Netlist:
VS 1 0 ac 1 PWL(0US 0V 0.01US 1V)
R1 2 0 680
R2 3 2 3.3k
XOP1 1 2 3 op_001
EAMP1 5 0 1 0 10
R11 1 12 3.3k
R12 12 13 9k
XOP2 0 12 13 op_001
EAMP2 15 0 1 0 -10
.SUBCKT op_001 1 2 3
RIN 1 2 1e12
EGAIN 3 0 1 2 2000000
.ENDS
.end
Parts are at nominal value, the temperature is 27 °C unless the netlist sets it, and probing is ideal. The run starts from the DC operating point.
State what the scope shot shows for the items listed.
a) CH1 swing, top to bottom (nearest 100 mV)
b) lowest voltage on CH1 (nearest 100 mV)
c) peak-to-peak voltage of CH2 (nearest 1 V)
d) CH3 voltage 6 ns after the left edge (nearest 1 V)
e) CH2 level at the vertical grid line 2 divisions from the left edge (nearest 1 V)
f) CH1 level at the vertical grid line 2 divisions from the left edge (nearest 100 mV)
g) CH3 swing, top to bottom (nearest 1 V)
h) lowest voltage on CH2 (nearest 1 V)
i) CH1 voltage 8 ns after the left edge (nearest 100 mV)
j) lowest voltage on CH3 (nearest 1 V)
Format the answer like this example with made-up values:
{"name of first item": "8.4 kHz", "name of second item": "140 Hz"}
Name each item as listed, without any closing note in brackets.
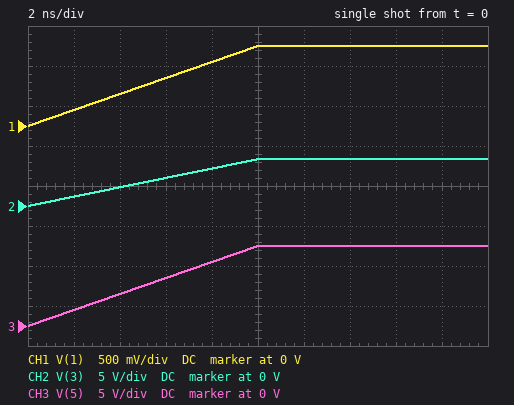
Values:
{"CH1 swing, top to bottom": "1.0 V", "lowest voltage on CH1": "0 V", "peak-to-peak voltage of CH2": "6 V", "CH3 voltage 6 ns after the left edge": "6 V", "CH2 level at the vertical grid line 2 divisions from the left edge": "2 V", "CH1 level at the vertical grid line 2 divisions from the left edge": "400 mV", "CH3 swing, top to bottom": "10 V", "lowest voltage on CH2": "0 V", "CH1 voltage 8 ns after the left edge": "800 mV", "lowest voltage on CH3": "0 V"}
